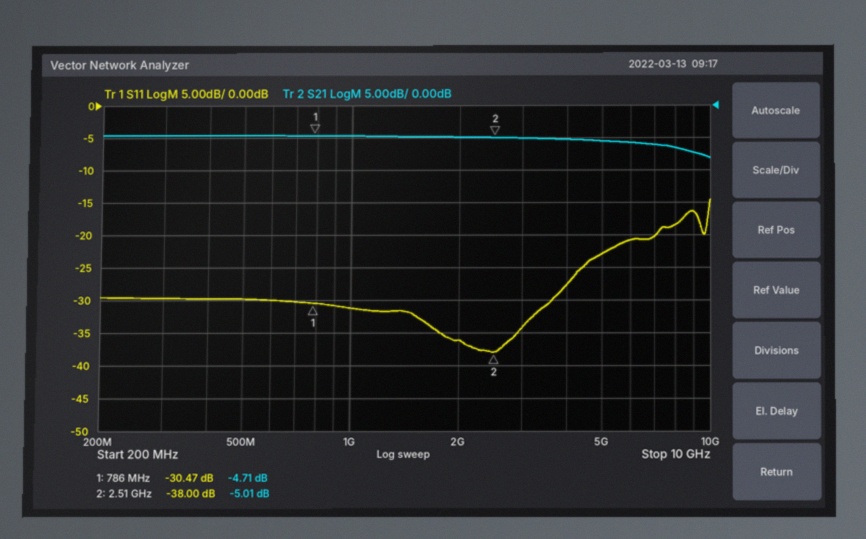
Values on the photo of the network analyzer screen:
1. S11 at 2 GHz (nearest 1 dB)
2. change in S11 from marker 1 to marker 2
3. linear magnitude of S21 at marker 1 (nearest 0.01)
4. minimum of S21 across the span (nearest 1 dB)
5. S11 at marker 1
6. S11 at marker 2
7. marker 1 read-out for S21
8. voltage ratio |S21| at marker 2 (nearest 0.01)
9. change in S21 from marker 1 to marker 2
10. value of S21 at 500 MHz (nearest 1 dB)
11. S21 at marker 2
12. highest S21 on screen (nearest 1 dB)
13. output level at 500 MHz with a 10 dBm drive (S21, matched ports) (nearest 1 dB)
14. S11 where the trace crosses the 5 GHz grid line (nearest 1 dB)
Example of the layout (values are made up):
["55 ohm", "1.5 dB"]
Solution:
["-36 dB", "-7.53 dB", "0.58", "-8 dB", "-30.47 dB", "-38.00 dB", "-4.71 dB", "0.56", "-0.30 dB", "-5 dB", "-5.01 dB", "-5 dB", "5 dBm", "-23 dB"]
